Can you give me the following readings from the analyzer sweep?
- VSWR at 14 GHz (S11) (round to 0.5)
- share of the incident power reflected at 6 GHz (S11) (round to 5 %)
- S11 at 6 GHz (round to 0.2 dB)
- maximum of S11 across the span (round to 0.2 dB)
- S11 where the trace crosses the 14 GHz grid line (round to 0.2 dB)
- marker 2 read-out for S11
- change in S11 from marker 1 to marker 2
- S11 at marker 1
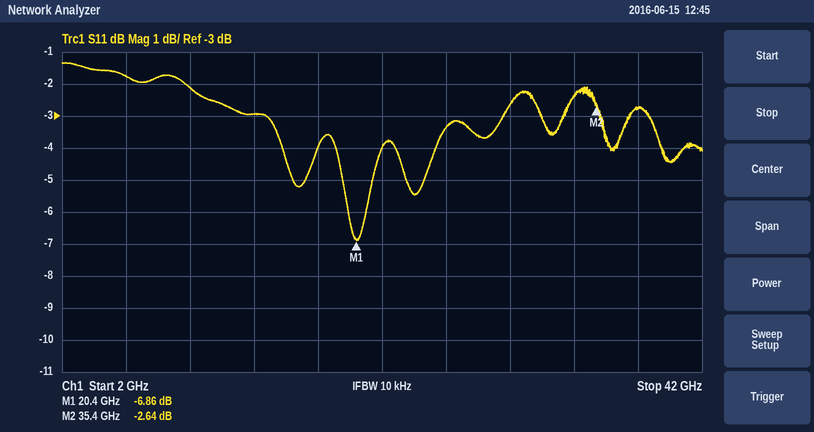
6.0
65 %
-1.8 dB
-1.4 dB
-3.0 dB
-2.64 dB
4.22 dB
-6.86 dB
